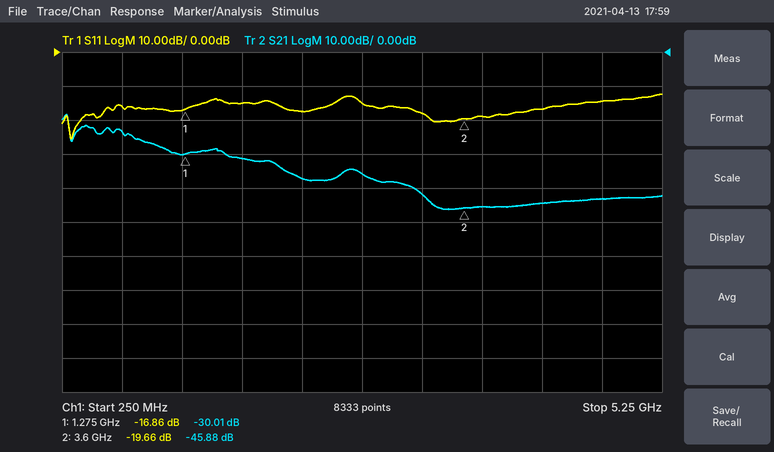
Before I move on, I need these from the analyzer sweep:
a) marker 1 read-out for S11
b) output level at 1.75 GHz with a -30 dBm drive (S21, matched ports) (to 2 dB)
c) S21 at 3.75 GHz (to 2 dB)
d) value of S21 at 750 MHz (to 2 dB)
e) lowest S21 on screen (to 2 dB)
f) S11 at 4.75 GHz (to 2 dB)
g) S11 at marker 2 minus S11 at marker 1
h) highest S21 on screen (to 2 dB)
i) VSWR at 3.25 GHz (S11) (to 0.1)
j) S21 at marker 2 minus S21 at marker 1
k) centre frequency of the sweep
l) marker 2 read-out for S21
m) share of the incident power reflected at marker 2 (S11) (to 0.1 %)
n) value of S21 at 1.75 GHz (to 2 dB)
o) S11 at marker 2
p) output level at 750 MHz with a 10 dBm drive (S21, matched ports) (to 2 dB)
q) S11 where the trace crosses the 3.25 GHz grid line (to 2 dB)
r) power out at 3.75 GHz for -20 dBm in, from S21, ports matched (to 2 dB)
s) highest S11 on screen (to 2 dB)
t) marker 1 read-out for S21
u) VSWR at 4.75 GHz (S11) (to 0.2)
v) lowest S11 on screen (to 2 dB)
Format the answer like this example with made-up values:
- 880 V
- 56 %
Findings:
- -16.86 dB
- -62 dBm
- -46 dB
- -24 dB
- -46 dB
- -14 dB
- -2.80 dB
- -18 dB
- 1.3
- -15.87 dB
- 2.75 GHz
- -45.88 dB
- 1.1 %
- -32 dB
- -19.66 dB
- -14 dBm
- -18 dB
- -66 dBm
- -12 dB
- -30.01 dB
- 1.4
- -26 dB
